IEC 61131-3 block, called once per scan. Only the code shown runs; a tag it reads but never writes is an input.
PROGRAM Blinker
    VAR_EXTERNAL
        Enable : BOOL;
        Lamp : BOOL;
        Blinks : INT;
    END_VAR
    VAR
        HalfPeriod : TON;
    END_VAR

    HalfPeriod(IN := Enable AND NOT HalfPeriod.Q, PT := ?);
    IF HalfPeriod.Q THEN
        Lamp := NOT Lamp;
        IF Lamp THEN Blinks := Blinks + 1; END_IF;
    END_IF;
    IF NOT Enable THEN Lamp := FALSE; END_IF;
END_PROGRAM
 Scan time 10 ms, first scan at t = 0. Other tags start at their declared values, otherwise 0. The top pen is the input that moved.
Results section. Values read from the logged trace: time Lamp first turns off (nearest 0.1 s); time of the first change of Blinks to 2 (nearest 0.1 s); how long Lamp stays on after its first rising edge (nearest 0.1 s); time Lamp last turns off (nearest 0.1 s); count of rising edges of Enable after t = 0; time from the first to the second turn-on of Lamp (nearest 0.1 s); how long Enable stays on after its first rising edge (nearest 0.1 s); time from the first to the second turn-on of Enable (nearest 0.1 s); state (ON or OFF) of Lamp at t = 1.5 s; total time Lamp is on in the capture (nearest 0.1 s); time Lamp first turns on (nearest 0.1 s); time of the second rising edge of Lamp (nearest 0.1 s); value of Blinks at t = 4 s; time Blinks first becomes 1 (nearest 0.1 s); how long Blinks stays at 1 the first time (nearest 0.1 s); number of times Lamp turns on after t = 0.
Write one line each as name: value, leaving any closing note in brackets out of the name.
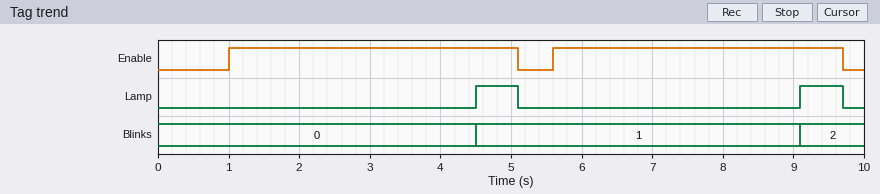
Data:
time Lamp first turns off: 5.1 s
time of the first change of Blinks to 2: 9.1 s
how long Lamp stays on after its first rising edge: 0.6 s
time Lamp last turns off: 9.7 s
count of rising edges of Enable after t = 0: 2
time from the first to the second turn-on of Lamp: 4.6 s
how long Enable stays on after its first rising edge: 4.1 s
time from the first to the second turn-on of Enable: 4.6 s
state (ON or OFF) of Lamp at t = 1.5 s: OFF
total time Lamp is on in the capture: 1.2 s
time Lamp first turns on: 4.5 s
time of the second rising edge of Lamp: 9.1 s
value of Blinks at t = 4 s: 0
time Blinks first becomes 1: 4.5 s
how long Blinks stays at 1 the first time: 4.6 s
number of times Lamp turns on after t = 0: 2
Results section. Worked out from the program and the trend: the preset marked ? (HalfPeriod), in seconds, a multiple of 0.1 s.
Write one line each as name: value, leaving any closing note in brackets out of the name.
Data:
the preset marked ? (HalfPeriod), in seconds, a multiple of 0.1 s: 3.5 s
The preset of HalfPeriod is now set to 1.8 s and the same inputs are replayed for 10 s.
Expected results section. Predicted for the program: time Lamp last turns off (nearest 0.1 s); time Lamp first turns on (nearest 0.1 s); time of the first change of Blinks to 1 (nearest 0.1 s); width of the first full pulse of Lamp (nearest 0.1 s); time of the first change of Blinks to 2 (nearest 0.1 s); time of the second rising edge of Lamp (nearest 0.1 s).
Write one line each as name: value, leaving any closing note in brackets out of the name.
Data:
time Lamp last turns off: 9.2 s
time Lamp first turns on: 2.8 s
time of the first change of Blinks to 1: 2.8 s
width of the first full pulse of Lamp: 1.8 s
time of the first change of Blinks to 2: 7.4 s
time of the second rising edge of Lamp: 7.4 s
